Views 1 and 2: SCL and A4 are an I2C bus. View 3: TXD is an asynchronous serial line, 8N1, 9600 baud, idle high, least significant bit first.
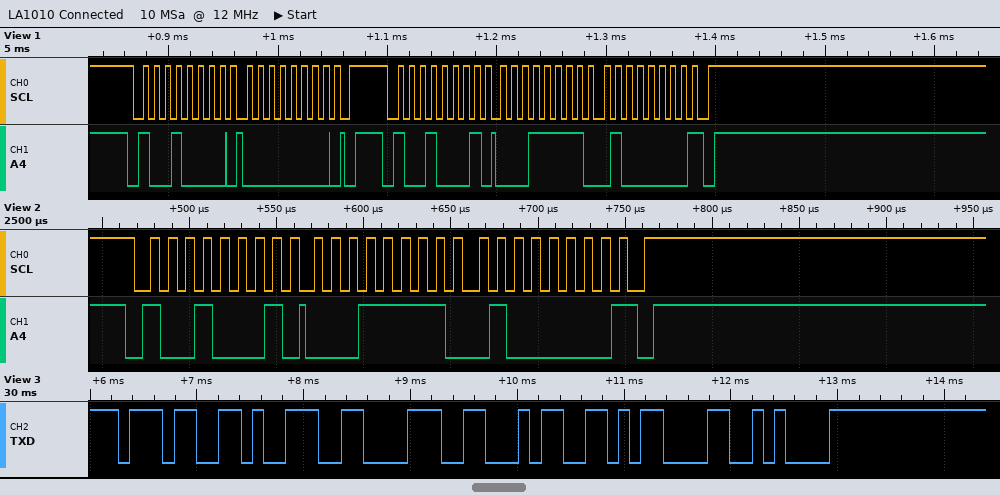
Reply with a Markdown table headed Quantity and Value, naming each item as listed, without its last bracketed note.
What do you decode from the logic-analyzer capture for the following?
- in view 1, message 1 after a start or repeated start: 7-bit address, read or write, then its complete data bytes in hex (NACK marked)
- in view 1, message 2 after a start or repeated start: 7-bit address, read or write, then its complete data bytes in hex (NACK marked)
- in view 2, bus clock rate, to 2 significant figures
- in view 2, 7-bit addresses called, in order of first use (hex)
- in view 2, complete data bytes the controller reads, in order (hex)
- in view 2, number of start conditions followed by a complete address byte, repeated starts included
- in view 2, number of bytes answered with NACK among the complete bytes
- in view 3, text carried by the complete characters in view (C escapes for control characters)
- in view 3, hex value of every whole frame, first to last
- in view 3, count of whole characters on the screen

| Quantity | Value |
|---|---|
| in view 1, message 1 after a start or repeated start: 7-bit address, read or write, then its complete data bytes in hex | 0x48 write: 00 |
| in view 1, message 2 after a start or repeated start: 7-bit address, read or write, then its complete data bytes in hex | 0x48 read: 1F 40 NACK |
| in view 2, bus clock rate, to 2 significant figures | 100 kHz |
| in view 2, 7-bit addresses called, in order of first use | 0x48 |
| in view 2, complete data bytes the controller reads, in order | 1F 40 |
| in view 2, number of start conditions followed by a complete address byte, repeated starts included | 1 |
| in view 2, number of bytes answered with NACK among the complete bytes | 1 |
| in view 3, text carried by the complete characters in view | "7984\r\n" |
| in view 3, hex value of every whole frame, first to last | 37 39 38 34 0D 0A |
| in view 3, count of whole characters on the screen | 6 |
